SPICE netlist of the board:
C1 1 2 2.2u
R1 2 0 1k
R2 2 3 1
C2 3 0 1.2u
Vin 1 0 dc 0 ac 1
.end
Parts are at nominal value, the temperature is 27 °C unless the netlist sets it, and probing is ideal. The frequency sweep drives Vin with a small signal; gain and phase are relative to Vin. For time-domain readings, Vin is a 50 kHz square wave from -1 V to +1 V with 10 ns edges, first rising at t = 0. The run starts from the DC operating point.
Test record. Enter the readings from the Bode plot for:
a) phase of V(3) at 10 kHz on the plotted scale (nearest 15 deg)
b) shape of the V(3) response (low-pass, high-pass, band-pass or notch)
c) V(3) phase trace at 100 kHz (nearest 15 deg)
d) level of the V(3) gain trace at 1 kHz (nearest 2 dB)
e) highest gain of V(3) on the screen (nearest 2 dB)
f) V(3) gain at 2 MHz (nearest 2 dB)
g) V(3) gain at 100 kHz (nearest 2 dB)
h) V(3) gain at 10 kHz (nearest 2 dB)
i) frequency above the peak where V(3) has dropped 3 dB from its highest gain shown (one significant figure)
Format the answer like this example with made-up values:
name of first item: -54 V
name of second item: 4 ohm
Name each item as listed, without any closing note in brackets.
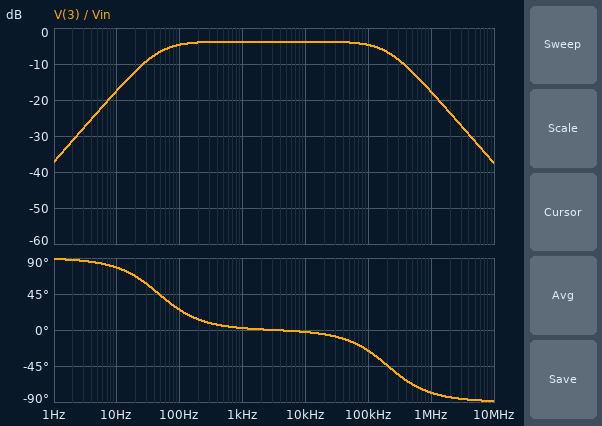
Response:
phase of V(3) at 10 kHz on the plotted scale: 0 deg
shape of the V(3) response: band-pass
V(3) phase trace at 100 kHz: -30 deg
level of the V(3) gain trace at 1 kHz: -4 dB
highest gain of V(3) on the screen: -4 dB
V(3) gain at 2 MHz: -24 dB
V(3) gain at 100 kHz: -4 dB
V(3) gain at 10 kHz: -4 dB
frequency above the peak where V(3) has dropped 3 dB from its highest gain shown: 200 kHz
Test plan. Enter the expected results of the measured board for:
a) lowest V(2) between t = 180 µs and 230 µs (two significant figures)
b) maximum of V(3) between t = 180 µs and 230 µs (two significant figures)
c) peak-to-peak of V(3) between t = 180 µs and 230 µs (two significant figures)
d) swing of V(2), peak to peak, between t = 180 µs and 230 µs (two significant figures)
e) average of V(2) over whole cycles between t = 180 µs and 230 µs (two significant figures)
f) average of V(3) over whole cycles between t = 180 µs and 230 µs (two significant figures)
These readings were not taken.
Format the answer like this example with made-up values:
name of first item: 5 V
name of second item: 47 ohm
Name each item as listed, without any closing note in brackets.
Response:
lowest V(2) between t = 180 µs and 230 µs: -740 mV
maximum of V(3) between t = 180 µs and 230 µs: 1.3 V
peak-to-peak of V(3) between t = 180 µs and 230 µs: 1.3 V
swing of V(2), peak to peak, between t = 180 µs and 230 µs: 2.7 V
average of V(2) over whole cycles between t = 180 µs and 230 µs: 610 mV
average of V(3) over whole cycles between t = 180 µs and 230 µs: 610 mV
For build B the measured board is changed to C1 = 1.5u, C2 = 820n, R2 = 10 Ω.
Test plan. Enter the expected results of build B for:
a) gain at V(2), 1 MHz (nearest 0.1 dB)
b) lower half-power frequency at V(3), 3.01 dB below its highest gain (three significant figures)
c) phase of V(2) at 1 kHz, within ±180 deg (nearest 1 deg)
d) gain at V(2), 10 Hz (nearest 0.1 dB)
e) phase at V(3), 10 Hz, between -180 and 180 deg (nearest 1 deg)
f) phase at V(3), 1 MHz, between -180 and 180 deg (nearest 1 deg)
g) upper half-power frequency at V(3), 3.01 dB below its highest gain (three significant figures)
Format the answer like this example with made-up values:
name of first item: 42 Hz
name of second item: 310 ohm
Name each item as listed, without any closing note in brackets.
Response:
gain at V(2), 1 MHz: 0 dB
lower half-power frequency at V(3), 3.01 dB below its highest gain: 68.2 Hz
phase of V(2) at 1 kHz, within ±180 deg: 5 deg
gain at V(2), 10 Hz: -20.6 dB
phase at V(3), 10 Hz, between -180 and 180 deg: 82 deg
phase at V(3), 1 MHz, between -180 and 180 deg: -88 deg
upper half-power frequency at V(3), 3.01 dB below its highest gain: 30.2 kHz
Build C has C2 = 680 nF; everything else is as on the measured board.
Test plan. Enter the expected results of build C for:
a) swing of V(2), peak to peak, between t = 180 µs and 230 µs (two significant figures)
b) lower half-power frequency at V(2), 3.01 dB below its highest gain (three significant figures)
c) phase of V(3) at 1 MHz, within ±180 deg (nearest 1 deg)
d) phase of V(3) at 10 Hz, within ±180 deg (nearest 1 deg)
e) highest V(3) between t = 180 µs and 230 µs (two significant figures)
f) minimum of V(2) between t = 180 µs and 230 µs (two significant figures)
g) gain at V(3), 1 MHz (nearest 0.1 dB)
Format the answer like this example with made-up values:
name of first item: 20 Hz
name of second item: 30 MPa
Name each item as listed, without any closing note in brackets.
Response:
swing of V(2), peak to peak, between t = 180 µs and 230 µs: 2.5 V
lower half-power frequency at V(2), 3.01 dB below its highest gain: 135 Hz
phase of V(3) at 1 MHz, within ±180 deg: -73 deg
phase of V(3) at 10 Hz, within ±180 deg: 80 deg
highest V(3) between t = 180 µs and 230 µs: 1.5 V
minimum of V(2) between t = 180 µs and 230 µs: -520 mV
gain at V(3), 1 MHz: -13.0 dB
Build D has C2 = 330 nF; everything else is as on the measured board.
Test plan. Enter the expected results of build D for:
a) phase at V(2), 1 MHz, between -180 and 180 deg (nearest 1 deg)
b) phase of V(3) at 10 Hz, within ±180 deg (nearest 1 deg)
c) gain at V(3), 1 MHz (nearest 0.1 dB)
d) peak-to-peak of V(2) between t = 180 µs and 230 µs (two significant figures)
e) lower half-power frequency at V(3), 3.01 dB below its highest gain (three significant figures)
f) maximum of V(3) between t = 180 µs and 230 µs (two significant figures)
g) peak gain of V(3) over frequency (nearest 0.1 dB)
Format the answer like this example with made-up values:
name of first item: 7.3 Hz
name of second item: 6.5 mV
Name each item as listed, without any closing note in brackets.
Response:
phase at V(2), 1 MHz, between -180 and 180 deg: 3 deg
phase of V(3) at 10 Hz, within ±180 deg: 81 deg
gain at V(3), 1 MHz: -7.5 dB
peak-to-peak of V(2) between t = 180 µs and 230 µs: 2.3 V
lower half-power frequency at V(3), 3.01 dB below its highest gain: 62.9 Hz
maximum of V(3) between t = 180 µs and 230 µs: 1.7 V
peak gain of V(3) over frequency: -1.2 dB
